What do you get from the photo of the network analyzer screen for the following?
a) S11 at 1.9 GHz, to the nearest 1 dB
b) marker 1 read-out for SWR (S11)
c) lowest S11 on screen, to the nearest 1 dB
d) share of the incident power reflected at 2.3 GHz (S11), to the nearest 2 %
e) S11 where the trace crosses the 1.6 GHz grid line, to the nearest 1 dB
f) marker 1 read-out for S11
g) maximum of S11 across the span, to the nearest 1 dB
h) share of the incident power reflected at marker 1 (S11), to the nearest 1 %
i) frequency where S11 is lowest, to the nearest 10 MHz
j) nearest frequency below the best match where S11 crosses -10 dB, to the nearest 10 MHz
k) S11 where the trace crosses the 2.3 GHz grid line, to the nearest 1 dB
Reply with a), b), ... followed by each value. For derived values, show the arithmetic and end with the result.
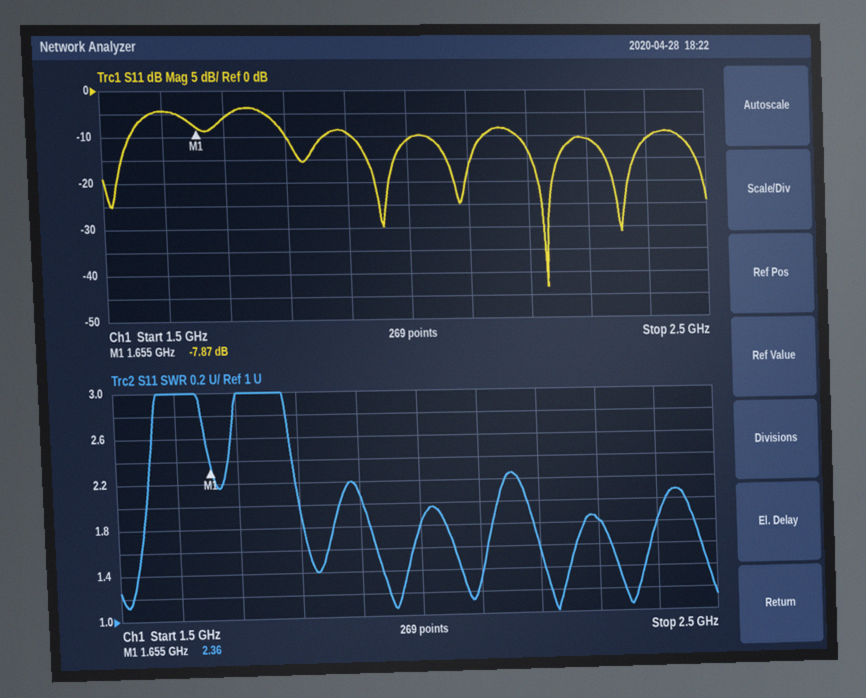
a) -9 dB
b) 2.36
c) -43 dB
d) 10^(-11/10) ≈ 8 %
e) -4 dB
f) -7.87 dB
g) -4 dB
h) 10^(-7.87/10) ≈ 16 %
i) 2.23 GHz
j) 2.18 GHz
k) -11 dB
